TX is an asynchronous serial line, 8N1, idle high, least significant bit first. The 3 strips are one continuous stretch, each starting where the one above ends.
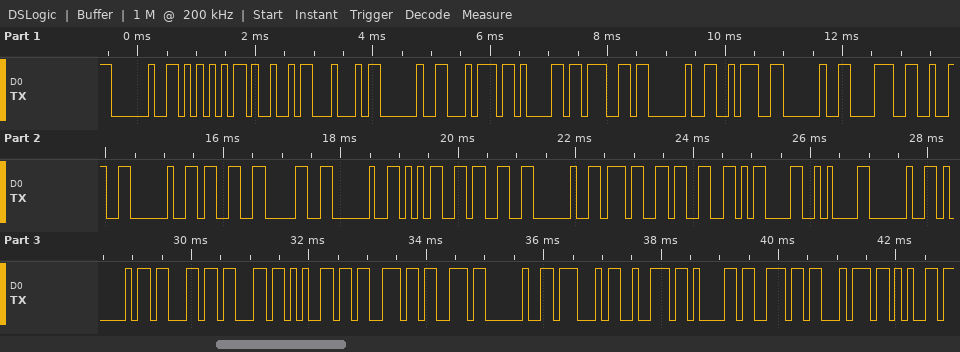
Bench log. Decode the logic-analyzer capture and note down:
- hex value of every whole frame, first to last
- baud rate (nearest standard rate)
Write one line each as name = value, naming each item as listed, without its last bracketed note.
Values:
hex value of every whole frame, first to last = 20 55 49 44 20 74 61 67 20 3A 20 38 32 20 33 30 20 35 33 20 37 33 0D 0A 20 41 63 63 65 73 73 20 47 72 61 6E 74 65
baud rate = 9600 baud
